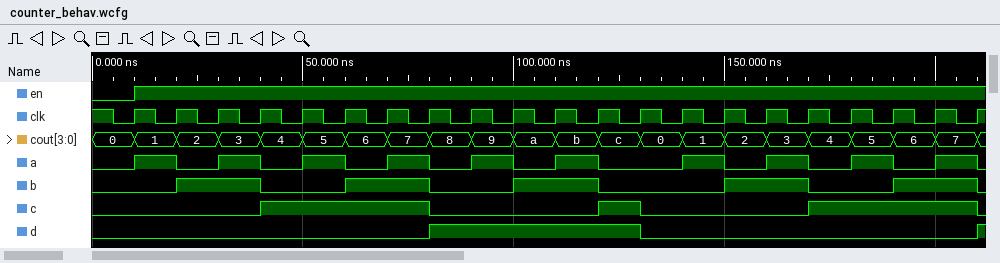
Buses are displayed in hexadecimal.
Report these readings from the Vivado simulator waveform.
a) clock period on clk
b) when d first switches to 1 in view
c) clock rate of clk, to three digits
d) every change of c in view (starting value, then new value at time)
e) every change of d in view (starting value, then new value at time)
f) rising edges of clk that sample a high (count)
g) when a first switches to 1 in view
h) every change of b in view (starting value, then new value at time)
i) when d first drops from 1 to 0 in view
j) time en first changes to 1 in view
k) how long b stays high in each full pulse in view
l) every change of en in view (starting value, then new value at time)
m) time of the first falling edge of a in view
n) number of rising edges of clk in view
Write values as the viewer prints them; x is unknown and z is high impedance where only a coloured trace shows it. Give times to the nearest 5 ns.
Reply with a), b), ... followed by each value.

a) 10 ns
b) 80 ns
c) 100 MHz
d) 0, 1 at 40 ns, 0 at 80 ns, 1 at 120 ns, 0 at 130 ns, 1 at 170 ns, 0 at 210 ns
e) 0, 1 at 80 ns, 0 at 130 ns, 1 at 210 ns
f) 10
g) 10 ns
h) 0, 1 at 20 ns, 0 at 40 ns, 1 at 60 ns, 0 at 80 ns, 1 at 100 ns, 0 at 120 ns, 1 at 150 ns, 0 at 170 ns, 1 at 190 ns, 0 at 210 ns
i) 130 ns
j) 10 ns
k) 20 ns, 20 ns, 20 ns, 20 ns, 20 ns
l) 0, 1 at 10 ns
m) 20 ns
n) 21
